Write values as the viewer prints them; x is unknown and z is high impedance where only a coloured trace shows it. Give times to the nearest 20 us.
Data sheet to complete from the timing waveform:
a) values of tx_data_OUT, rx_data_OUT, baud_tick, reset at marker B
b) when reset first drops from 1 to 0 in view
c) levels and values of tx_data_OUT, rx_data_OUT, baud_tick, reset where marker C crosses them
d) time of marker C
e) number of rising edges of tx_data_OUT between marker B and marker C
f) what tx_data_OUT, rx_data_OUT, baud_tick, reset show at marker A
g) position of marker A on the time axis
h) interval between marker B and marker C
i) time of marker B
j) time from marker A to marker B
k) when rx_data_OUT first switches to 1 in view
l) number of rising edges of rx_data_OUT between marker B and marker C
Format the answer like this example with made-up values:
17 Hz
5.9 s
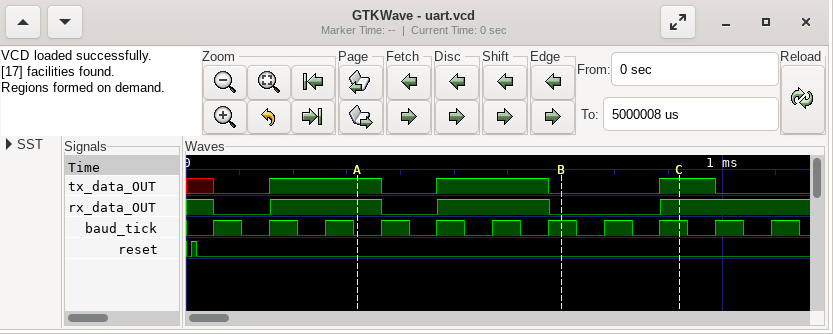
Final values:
tx_data_OUT=0, rx_data_OUT=0, baud_tick=1, reset=0
20 us
tx_data_OUT=1, rx_data_OUT=1, baud_tick=1, reset=0
920 us
1
tx_data_OUT=1, rx_data_OUT=1, baud_tick=0, reset=0
320 us
220 us
700 us
380 us
160 us
1
